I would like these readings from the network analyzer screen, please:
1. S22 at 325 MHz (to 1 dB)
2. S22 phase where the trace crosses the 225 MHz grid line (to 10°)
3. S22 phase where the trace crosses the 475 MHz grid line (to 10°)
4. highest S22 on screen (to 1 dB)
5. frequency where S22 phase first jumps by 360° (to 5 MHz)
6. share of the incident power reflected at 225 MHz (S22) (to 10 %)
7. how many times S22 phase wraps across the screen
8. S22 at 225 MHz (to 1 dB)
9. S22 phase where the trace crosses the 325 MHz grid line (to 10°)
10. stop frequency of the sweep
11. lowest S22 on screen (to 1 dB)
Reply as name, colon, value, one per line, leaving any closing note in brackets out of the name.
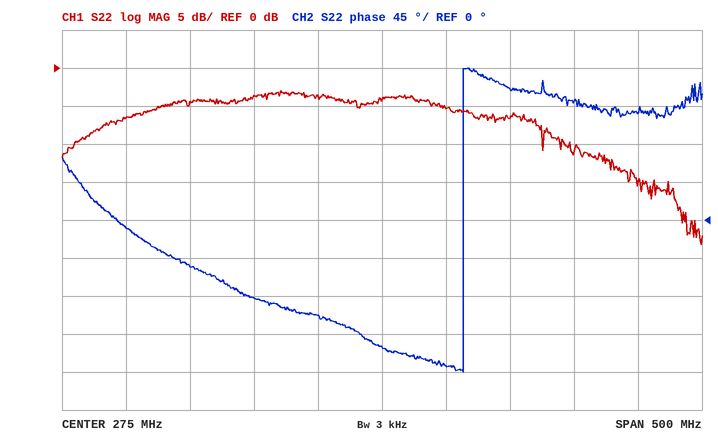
S22 at 325 MHz: -5 dB
S22 phase where the trace crosses the 225 MHz grid line: -110°
S22 phase where the trace crosses the 475 MHz grid line: 130°
highest S22 on screen: -3 dB
frequency where S22 phase first jumps by 360°: 340 MHz
share of the incident power reflected at 225 MHz (S22): 40 %
how many times S22 phase wraps across the screen: 1
S22 at 225 MHz: -4 dB
S22 phase where the trace crosses the 325 MHz grid line: -170°
stop frequency of the sweep: 525 MHz
lowest S22 on screen: -23 dB
